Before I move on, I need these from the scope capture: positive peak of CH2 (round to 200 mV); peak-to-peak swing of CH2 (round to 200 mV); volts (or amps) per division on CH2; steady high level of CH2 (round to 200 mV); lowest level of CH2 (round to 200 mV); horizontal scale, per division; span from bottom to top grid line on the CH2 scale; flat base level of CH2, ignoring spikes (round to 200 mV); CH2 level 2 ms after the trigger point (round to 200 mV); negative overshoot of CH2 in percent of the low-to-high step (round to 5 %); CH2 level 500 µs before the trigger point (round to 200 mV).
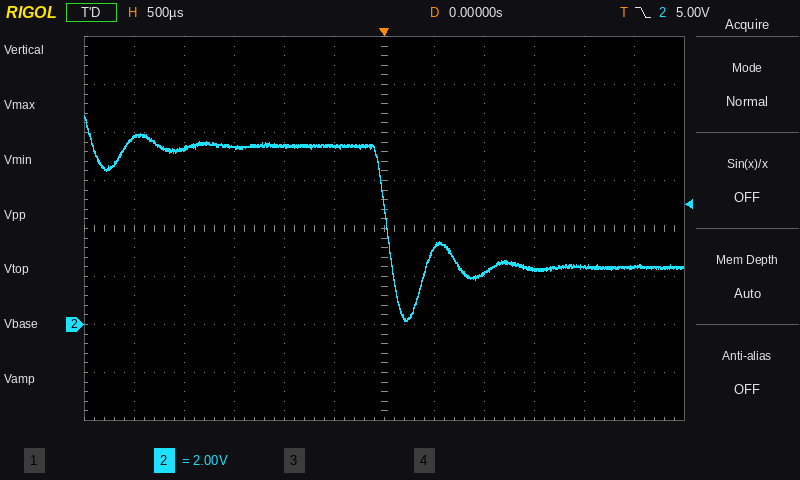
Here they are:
8.8 V
8.6 V
2 V
7.4 V
200 mV
500 µs
16 V
2.4 V
2.4 V
45 %
7.4 V
